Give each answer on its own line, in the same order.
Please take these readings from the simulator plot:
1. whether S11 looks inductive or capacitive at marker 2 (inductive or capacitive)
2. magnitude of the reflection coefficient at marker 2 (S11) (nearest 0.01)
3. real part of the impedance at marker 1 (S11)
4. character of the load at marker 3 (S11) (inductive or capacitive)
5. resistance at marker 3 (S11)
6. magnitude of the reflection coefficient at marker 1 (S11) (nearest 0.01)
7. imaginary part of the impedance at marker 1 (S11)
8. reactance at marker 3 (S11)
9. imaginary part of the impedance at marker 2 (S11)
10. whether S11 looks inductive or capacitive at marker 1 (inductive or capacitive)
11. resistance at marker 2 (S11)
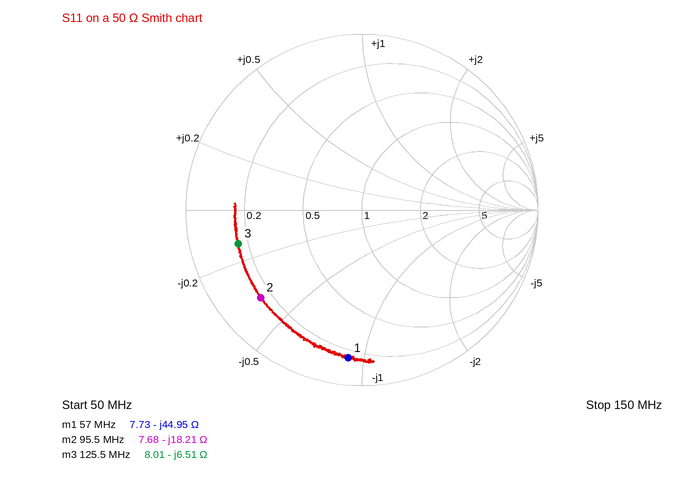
capacitive
0.76
7.73 Ω
capacitive
8.01 Ω
0.84
-44.95 Ω
-6.51 Ω
-18.21 Ω
capacitive
7.68 Ω
